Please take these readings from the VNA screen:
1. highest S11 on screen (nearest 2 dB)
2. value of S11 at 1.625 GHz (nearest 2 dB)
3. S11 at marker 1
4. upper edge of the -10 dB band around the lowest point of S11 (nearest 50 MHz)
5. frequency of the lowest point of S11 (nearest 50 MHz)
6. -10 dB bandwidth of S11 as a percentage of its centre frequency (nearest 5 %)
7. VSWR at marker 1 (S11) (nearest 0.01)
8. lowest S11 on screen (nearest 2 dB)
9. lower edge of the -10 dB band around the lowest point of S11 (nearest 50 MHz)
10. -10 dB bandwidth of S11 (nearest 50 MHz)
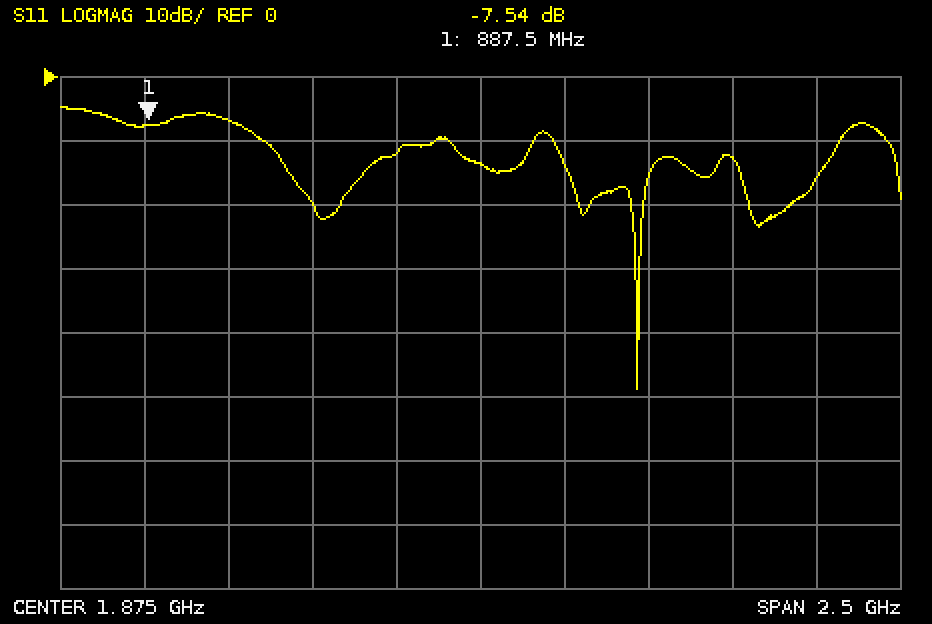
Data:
-4 dB
-12 dB
-7.54 dB
2.95 GHz
2.35 GHz
35 %
2.45
-48 dB
2.10 GHz
850 MHz
